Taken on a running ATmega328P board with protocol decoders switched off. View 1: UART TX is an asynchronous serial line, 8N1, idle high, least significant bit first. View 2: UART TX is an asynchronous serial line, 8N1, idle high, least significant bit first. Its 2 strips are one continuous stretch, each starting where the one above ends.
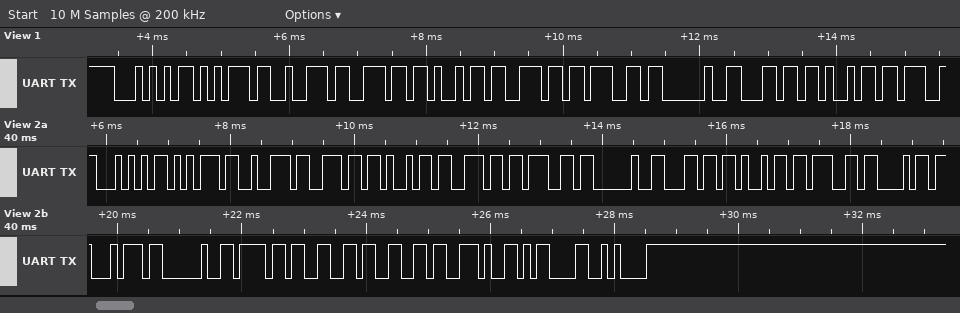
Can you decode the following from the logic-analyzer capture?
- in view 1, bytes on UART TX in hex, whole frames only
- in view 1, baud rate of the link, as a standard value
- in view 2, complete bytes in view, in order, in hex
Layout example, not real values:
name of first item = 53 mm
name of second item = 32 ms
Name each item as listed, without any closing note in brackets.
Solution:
in view 1, bytes on UART TX in hex, whole frames only = 54 75 72 6E 69 6E 67 20 6C 69
in view 1, baud rate of the link, as a standard value = 9600 baud
in view 2, complete bytes in view, in order, in hex = 54 75 72 6E 69 6E 67 20 6C 69 67 68 74 20 6F 66 66 2E 0D 0A
